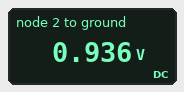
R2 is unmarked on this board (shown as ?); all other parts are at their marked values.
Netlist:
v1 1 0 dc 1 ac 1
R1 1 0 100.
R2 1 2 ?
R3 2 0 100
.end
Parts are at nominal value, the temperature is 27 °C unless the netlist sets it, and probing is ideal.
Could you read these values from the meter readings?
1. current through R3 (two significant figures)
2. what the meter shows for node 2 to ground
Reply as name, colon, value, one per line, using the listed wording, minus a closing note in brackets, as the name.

current through R3: 9.4 mA
what the meter shows for node 2 to ground: 0.936 V
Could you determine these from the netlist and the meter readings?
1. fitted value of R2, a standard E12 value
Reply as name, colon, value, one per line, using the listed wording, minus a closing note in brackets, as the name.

fitted value of R2, a standard E12 value: 6.8 Ω
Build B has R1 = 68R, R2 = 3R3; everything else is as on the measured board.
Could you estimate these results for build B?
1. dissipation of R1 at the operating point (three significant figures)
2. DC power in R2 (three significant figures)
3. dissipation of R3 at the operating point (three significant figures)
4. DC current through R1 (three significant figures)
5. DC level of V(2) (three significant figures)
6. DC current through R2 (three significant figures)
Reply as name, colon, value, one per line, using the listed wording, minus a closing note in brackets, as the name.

dissipation of R1 at the operating point: 14.7 mW
DC power in R2: 309 µW
dissipation of R3 at the operating point: 9.37 mW
DC current through R1: 14.7 mA
DC level of V(2): 968 mV
DC current through R2: 9.68 mA
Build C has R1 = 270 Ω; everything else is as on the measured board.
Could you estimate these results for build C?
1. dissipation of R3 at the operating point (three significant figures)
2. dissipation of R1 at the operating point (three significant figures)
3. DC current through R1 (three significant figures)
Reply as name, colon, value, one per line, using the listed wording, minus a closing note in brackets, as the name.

dissipation of R3 at the operating point: 8.77 mW
dissipation of R1 at the operating point: 3.70 mW
DC current through R1: 3.70 mA
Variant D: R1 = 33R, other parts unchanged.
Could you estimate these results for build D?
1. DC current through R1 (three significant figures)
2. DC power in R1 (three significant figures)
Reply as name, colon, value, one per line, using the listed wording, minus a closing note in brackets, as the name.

DC current through R1: 30.3 mA
DC power in R1: 30.3 mW
